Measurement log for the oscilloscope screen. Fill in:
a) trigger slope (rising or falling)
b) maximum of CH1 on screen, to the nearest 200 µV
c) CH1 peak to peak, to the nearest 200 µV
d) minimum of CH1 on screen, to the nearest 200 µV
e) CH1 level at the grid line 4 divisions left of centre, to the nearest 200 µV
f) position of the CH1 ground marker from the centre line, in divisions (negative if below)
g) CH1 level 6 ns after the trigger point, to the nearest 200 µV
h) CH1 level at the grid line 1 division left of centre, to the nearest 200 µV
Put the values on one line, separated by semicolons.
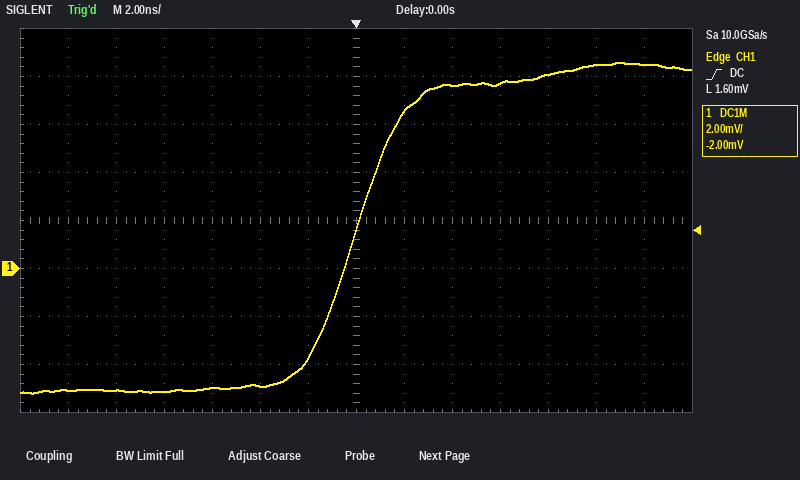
rising; 8.6 mV; 13.8 mV; -5.2 mV; -5.2 mV; -1.0 div; 7.8 mV; -3.8 mV
